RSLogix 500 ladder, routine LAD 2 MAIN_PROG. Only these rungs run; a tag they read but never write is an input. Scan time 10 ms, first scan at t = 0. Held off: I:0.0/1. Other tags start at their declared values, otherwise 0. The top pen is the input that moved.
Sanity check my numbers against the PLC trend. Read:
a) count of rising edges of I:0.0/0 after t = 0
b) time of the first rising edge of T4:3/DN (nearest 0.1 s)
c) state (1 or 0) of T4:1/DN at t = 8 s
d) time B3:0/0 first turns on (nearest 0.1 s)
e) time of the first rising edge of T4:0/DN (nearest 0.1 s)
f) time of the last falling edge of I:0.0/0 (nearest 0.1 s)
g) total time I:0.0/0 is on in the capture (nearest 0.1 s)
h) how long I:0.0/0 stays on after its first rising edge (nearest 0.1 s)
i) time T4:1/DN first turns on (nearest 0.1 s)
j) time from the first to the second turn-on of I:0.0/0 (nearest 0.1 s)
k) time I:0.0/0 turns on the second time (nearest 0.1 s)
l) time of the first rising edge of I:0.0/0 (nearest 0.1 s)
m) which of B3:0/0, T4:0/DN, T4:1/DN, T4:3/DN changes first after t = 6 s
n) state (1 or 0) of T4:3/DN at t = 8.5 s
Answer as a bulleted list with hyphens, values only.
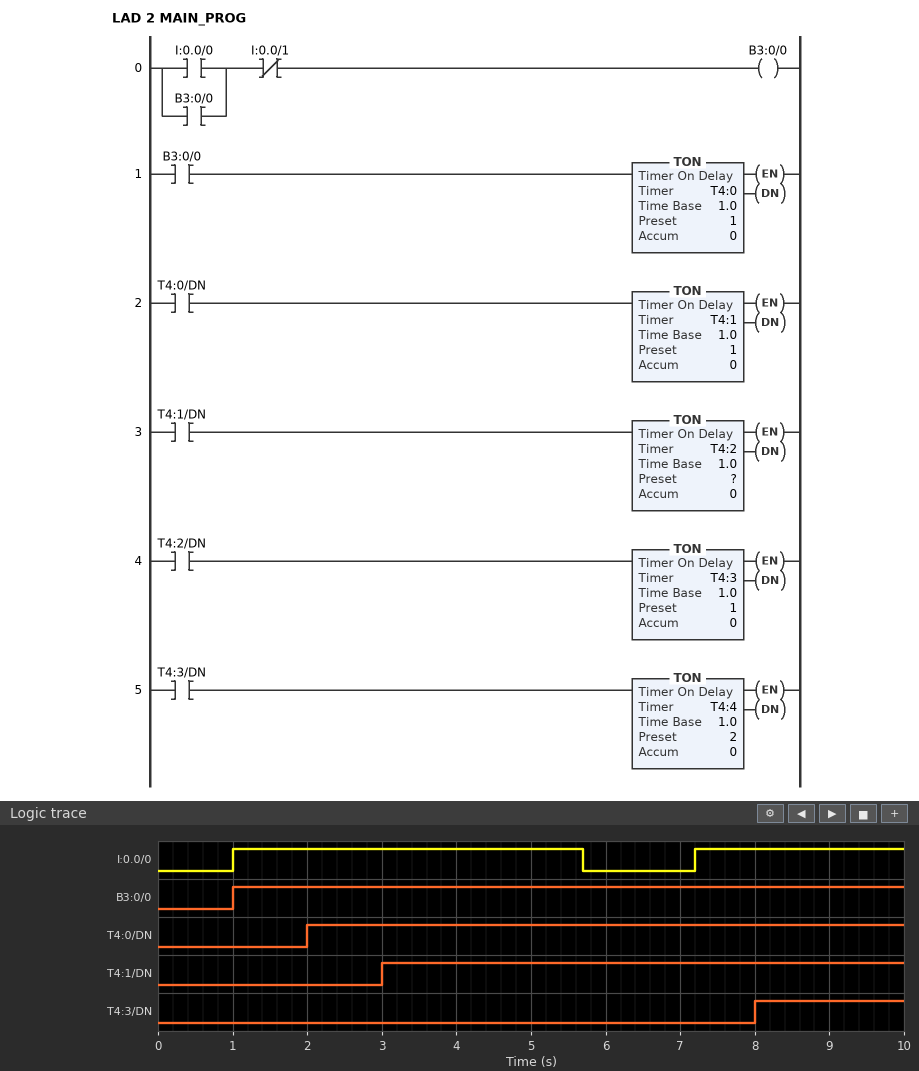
- 2
- 8.0 s
- 1
- 1.0 s
- 2.0 s
- 5.7 s
- 7.5 s
- 4.7 s
- 3.0 s
- 6.2 s
- 7.2 s
- 1.0 s
- T4:3/DN
- 1
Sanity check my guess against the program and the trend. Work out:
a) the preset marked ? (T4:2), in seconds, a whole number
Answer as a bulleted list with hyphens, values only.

- 4 s
